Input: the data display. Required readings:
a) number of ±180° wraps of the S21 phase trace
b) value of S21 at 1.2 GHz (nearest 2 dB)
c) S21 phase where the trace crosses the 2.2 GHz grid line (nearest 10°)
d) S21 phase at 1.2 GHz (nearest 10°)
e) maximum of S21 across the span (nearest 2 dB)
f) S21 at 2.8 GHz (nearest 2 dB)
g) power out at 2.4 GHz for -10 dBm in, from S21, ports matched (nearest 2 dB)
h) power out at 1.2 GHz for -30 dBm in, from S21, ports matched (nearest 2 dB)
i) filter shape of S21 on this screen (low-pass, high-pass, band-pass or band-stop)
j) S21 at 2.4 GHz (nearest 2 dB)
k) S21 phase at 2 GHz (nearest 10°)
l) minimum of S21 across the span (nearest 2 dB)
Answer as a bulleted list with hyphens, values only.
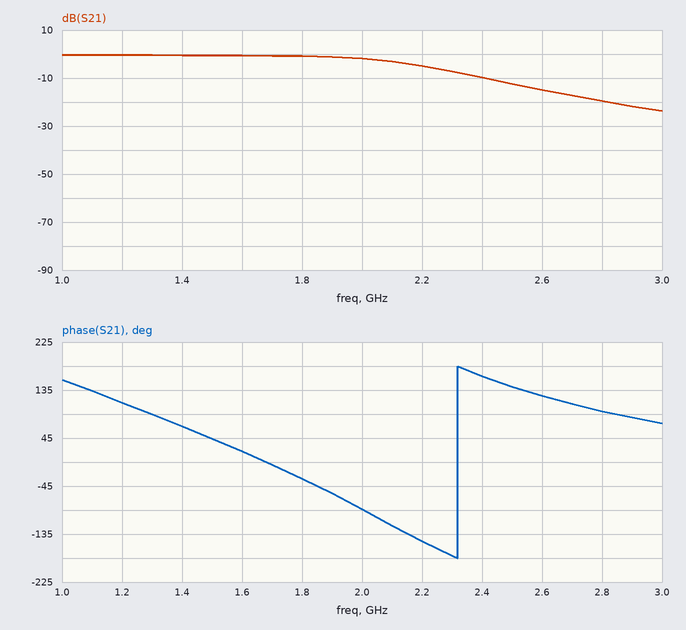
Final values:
- 1
- 0 dB
- -150°
- 110°
- 0 dB
- -20 dB
- -20 dBm
- -30 dBm
- low-pass
- -10 dB
- -90°
- -24 dB
